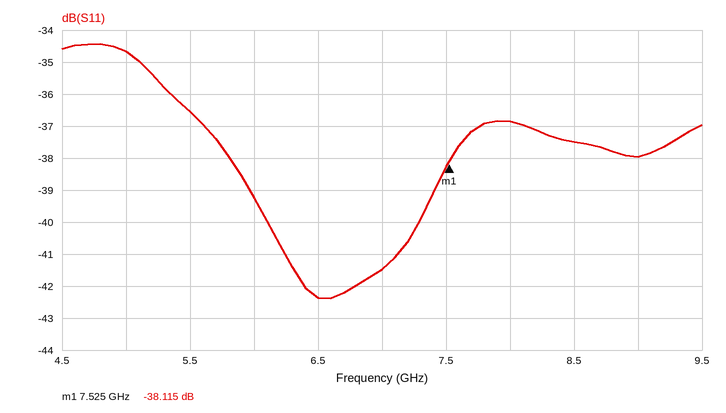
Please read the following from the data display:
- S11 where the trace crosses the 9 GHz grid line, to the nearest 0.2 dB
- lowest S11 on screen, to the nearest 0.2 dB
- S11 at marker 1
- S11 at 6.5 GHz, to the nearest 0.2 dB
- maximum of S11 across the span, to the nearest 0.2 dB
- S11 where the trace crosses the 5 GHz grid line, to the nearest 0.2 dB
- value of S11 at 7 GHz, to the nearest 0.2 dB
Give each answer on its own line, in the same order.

-38.0 dB
-42.4 dB
-38.115 dB
-42.4 dB
-34.4 dB
-34.6 dB
-41.4 dB
